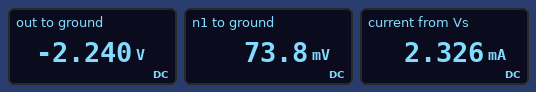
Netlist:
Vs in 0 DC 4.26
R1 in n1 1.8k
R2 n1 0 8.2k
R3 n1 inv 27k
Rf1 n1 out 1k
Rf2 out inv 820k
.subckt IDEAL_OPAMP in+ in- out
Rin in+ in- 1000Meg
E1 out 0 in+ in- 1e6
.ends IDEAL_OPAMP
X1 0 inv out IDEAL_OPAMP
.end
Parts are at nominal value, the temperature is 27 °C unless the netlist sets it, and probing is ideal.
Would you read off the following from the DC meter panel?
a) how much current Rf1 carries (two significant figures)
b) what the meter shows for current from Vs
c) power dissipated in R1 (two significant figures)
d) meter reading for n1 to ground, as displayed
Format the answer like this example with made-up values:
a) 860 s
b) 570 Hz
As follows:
a) 2.3 mA
b) 2.326 mA
c) 9.7 mW
d) 73.8 mV
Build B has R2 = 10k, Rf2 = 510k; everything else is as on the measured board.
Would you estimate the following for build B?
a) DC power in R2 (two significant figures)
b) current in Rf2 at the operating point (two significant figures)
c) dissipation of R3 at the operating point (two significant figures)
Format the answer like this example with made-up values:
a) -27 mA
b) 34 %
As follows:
a) 1.3 µW
b) 4.3 µA
c) 490 nW
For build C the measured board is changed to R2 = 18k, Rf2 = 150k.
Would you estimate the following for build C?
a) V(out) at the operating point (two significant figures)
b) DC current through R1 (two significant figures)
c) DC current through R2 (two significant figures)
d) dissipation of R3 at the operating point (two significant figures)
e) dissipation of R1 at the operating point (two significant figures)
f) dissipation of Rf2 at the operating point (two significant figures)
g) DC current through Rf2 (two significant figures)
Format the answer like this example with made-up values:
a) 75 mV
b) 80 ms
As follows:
a) -1.8 V
b) 2.2 mA
c) 18 µA
d) 4.0 µW
e) 8.6 mW
f) 22 µW
g) 12 µA
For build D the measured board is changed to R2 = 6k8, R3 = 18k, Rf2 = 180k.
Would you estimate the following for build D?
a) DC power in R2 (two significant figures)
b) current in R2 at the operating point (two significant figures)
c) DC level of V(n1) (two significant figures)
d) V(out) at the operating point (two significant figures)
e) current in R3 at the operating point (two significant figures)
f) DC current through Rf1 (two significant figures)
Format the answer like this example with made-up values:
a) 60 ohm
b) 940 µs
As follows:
a) 6.0 µW
b) 30 µA
c) 200 mV
d) -2.0 V
e) 11 µA
f) 2.2 mA
